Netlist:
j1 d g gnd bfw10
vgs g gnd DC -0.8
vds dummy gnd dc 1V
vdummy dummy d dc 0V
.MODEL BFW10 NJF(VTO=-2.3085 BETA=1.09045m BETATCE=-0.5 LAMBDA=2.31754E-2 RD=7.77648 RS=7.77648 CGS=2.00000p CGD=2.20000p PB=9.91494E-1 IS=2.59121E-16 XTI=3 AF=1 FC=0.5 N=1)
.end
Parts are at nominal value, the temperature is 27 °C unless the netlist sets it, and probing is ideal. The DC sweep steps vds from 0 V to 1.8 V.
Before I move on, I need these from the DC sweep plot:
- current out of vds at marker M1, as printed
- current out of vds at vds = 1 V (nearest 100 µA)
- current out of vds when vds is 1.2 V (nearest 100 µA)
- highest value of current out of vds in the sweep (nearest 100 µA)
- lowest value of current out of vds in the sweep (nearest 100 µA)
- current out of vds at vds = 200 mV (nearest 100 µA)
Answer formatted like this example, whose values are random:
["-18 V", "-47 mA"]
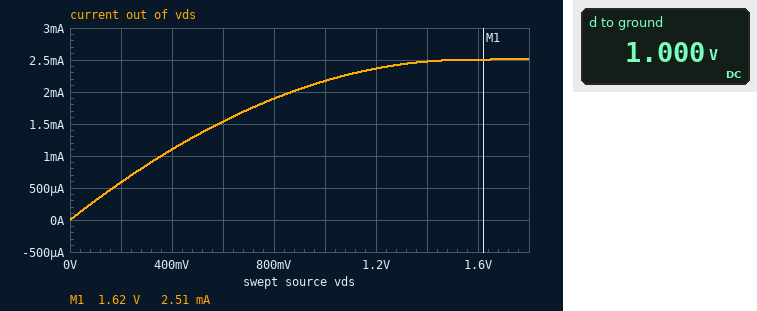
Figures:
["2.51 mA", "2.2 mA", "2.4 mA", "2.5 mA", "0 A", "600 µA"]
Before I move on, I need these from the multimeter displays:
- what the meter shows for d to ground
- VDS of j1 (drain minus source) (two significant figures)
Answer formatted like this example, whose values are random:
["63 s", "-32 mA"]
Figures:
["1.000 V", "1.0 V"]
